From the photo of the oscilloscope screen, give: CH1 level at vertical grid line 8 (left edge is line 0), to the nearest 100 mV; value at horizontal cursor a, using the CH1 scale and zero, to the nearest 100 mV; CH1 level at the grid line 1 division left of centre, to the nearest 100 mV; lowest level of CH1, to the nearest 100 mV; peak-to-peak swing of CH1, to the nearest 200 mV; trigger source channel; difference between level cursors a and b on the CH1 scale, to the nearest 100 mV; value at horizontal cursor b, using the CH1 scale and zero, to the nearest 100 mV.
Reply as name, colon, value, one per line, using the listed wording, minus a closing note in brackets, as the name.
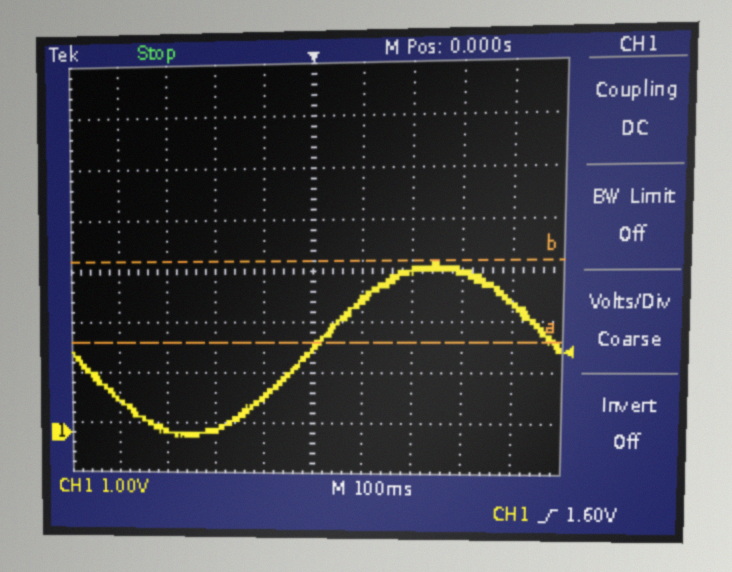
CH1 level at vertical grid line 8 (left edge is line 0), to the nearest 100 mV: 3.2 V
value at horizontal cursor a, using the CH1 scale and zero, to the nearest 100 mV: 1.8 V
CH1 level at the grid line 1 division left of centre, to the nearest 100 mV: 700 mV
lowest level of CH1, to the nearest 100 mV: -100 mV
peak-to-peak swing of CH1, to the nearest 200 mV: 3.4 V
trigger source channel: CH1
difference between level cursors a and b on the CH1 scale, to the nearest 100 mV: 1.6 V
value at horizontal cursor b, using the CH1 scale and zero, to the nearest 100 mV: 3.4 V
